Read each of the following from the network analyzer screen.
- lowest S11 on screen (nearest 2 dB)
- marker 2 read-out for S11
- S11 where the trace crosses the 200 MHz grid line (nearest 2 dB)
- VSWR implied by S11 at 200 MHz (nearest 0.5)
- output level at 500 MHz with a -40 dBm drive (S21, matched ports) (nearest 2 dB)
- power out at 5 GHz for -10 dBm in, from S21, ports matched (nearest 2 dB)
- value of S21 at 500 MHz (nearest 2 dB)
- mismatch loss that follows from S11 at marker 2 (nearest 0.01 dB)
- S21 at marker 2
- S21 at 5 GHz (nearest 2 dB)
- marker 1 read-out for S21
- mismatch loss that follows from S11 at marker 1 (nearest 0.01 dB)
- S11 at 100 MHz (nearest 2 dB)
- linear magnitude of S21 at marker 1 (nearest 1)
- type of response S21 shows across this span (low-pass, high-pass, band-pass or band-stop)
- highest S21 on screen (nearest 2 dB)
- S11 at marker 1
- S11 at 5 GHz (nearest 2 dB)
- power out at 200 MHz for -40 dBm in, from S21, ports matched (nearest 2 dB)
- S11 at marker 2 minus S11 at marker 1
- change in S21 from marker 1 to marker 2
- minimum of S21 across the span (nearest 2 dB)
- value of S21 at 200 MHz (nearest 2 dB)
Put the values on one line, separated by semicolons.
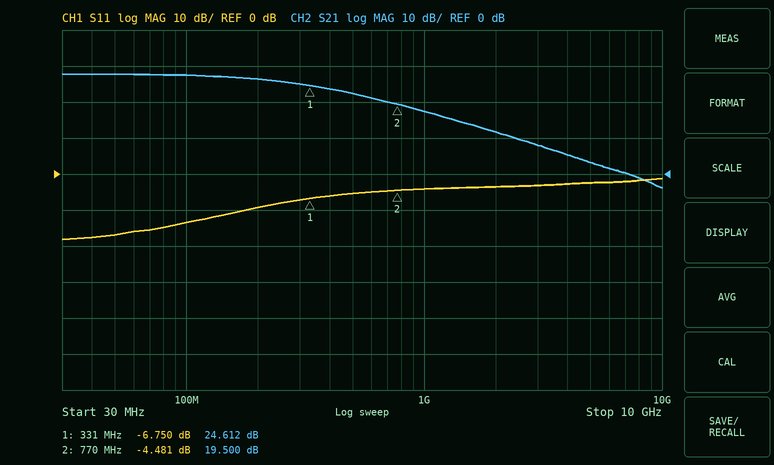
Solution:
-18 dB; -4.481 dB; -10 dB; 2.0; -18 dBm; -6 dBm; 22 dB; 1.91 dB; 19.500 dB; 4 dB; 24.612 dB; 1.03 dB; -14 dB; 17; low-pass; 28 dB; -6.750 dB; -2 dB; -14 dBm; 2.269 dB; -5.112 dB; -4 dB; 26 dB
